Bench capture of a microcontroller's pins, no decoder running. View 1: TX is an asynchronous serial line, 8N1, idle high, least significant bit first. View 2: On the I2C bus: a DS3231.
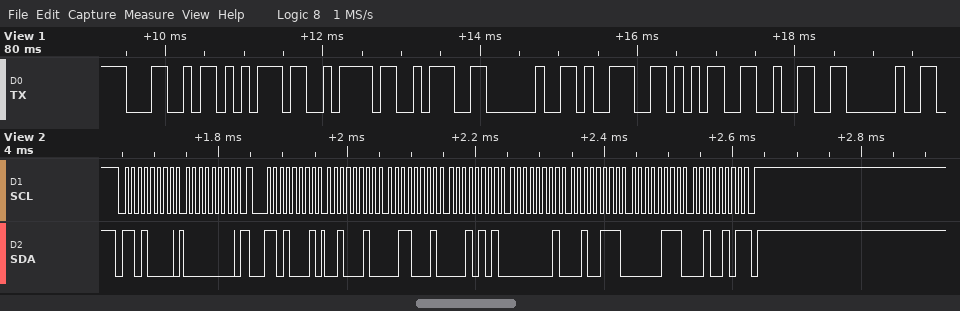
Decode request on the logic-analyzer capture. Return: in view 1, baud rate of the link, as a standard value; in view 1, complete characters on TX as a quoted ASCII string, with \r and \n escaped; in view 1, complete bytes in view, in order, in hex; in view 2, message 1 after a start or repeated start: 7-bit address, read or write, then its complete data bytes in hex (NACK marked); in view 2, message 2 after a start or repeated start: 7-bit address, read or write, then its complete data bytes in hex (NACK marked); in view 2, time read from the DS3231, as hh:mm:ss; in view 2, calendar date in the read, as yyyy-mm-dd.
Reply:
9600 baud
"Luz: 952 "
4C 75 7A 3A 20 39 35 32 20
0x68 write: 00
0x68 read: 22 31 15 01 27 07 25 NACK
15:31:22
2025-07-27
